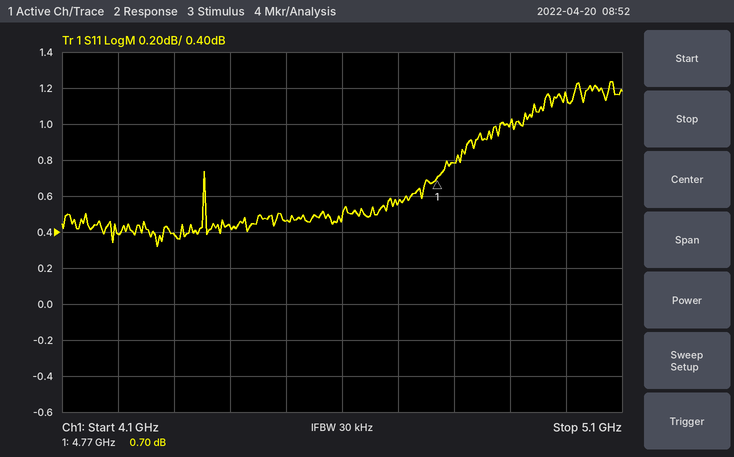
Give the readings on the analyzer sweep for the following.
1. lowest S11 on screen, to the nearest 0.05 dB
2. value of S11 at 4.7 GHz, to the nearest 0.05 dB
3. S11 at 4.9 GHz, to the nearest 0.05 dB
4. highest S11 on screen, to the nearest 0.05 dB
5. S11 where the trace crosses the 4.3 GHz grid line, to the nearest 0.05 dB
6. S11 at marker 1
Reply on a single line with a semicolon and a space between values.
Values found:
0.30 dB; 0.55 dB; 1.00 dB; 1.25 dB; 0.40 dB; 0.70 dB
